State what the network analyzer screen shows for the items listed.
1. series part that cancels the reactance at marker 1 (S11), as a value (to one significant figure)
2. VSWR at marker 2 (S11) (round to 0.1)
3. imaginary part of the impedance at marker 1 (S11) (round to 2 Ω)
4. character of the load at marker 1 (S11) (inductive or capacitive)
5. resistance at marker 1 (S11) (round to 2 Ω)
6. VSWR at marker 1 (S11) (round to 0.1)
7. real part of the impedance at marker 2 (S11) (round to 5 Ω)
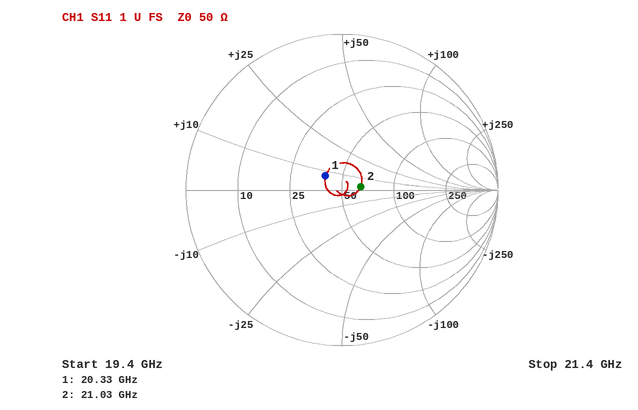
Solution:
1 pF
1.3
+8 Ω
inductive
40 Ω
1.3
65 Ω
